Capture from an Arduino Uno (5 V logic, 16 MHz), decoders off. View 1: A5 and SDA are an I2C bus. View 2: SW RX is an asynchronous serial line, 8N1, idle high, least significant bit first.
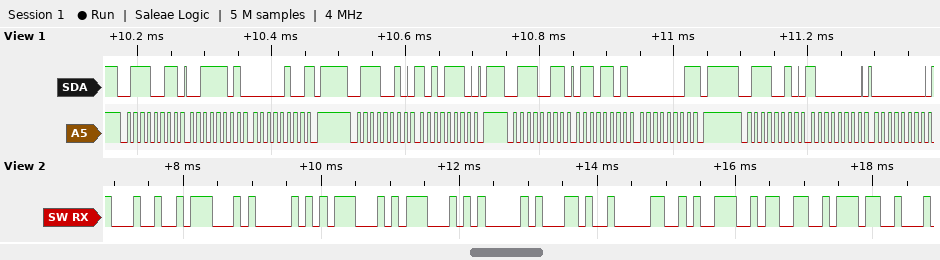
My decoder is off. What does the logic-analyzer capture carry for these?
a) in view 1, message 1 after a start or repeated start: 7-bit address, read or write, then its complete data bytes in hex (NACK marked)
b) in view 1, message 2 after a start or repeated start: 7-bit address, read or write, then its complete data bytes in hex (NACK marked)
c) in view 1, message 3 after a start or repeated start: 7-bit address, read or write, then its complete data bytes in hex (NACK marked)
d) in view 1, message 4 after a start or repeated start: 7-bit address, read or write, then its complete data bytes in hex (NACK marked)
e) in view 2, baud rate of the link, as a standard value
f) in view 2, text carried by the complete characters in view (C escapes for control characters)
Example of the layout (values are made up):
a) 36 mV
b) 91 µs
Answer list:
a) 0x39 read: 3D 04 NACK
b) 0x39 write: AE
c) 0x39 read: 6D 01 NACK
d) 0x39 write: 80 00
e) 9600 baud
f) "$GPGGA,0937"
